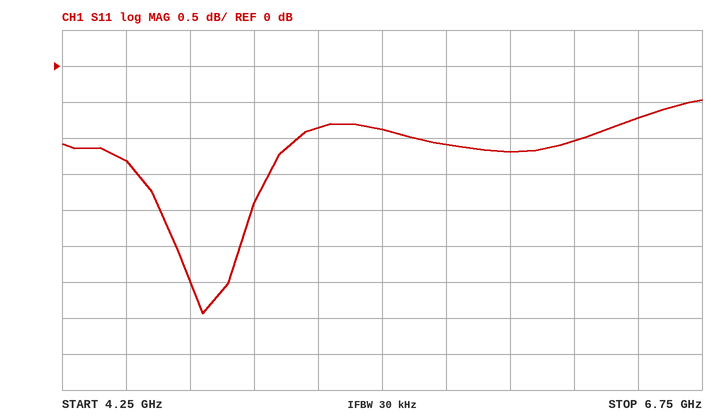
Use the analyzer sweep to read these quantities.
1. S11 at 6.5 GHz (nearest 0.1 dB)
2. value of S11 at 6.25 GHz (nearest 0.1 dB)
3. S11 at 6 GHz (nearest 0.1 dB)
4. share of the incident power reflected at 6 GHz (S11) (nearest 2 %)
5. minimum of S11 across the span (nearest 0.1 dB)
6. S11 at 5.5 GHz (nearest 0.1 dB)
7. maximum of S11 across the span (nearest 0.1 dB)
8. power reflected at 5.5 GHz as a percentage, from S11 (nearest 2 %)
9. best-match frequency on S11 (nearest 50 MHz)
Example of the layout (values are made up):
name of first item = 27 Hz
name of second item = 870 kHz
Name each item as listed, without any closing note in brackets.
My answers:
S11 at 6.5 GHz = -0.7 dB
value of S11 at 6.25 GHz = -1.0 dB
S11 at 6 GHz = -1.2 dB
share of the incident power reflected at 6 GHz (S11) = 76 %
minimum of S11 across the span = -3.4 dB
S11 at 5.5 GHz = -0.9 dB
maximum of S11 across the span = -0.5 dB
power reflected at 5.5 GHz as a percentage, from S11 = 82 %
best-match frequency on S11 = 4.80 GHz
